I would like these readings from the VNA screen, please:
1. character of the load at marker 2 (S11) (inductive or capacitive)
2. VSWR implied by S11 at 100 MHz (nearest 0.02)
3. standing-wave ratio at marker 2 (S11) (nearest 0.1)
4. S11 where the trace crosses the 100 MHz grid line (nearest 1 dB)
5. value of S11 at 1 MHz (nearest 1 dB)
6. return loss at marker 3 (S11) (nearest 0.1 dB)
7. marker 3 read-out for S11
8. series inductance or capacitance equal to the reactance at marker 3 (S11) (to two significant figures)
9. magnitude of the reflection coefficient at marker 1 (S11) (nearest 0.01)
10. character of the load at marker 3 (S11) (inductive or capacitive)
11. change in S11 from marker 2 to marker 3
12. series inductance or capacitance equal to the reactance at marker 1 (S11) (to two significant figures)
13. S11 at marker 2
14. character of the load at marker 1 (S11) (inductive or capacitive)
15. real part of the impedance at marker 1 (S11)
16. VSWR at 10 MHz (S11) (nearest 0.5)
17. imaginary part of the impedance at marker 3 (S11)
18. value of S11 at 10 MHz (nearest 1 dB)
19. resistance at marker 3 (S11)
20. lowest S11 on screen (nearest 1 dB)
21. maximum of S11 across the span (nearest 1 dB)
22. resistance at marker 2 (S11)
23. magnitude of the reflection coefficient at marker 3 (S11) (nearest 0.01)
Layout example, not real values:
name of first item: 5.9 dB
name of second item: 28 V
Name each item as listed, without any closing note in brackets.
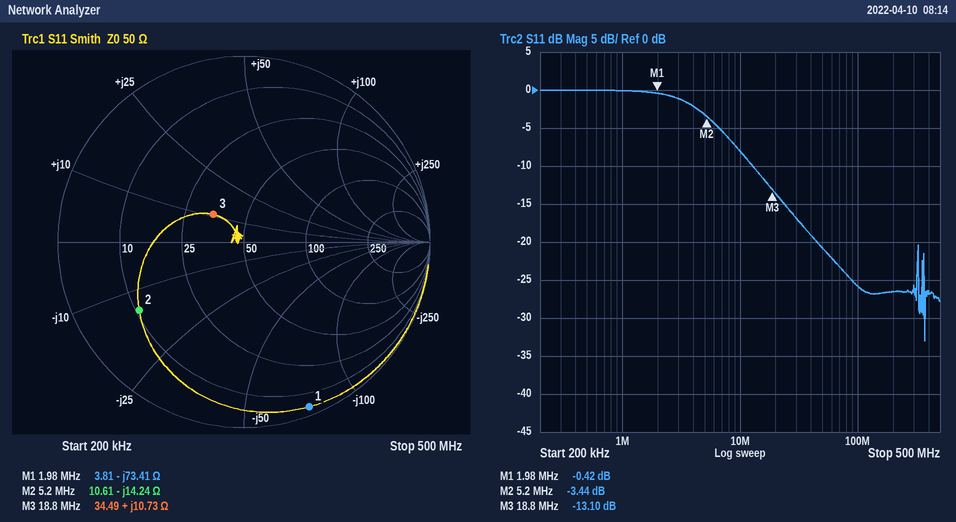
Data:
character of the load at marker 2 (S11): capacitive
VSWR implied by S11 at 100 MHz: 1.10
standing-wave ratio at marker 2 (S11): 5.1
S11 where the trace crosses the 100 MHz grid line: -26 dB
value of S11 at 1 MHz: 0 dB
return loss at marker 3 (S11): 13.1 dB
marker 3 read-out for S11: -13.10 dB
series inductance or capacitance equal to the reactance at marker 3 (S11): 91 nH
magnitude of the reflection coefficient at marker 1 (S11): 0.95
character of the load at marker 3 (S11): inductive
change in S11 from marker 2 to marker 3: -9.66 dB
series inductance or capacitance equal to the reactance at marker 1 (S11): 1.1 nF
S11 at marker 2: -3.44 dB
character of the load at marker 1 (S11): capacitive
real part of the impedance at marker 1: 3.81 Ω
VSWR at 10 MHz (S11): 2.5
imaginary part of the impedance at marker 3: +10.73 Ω
value of S11 at 10 MHz: -8 dB
resistance at marker 3: 34.49 Ω
lowest S11 on screen: -33 dB
maximum of S11 across the span: 0 dB
resistance at marker 2: 10.61 Ω
magnitude of the reflection coefficient at marker 3 (S11): 0.22
